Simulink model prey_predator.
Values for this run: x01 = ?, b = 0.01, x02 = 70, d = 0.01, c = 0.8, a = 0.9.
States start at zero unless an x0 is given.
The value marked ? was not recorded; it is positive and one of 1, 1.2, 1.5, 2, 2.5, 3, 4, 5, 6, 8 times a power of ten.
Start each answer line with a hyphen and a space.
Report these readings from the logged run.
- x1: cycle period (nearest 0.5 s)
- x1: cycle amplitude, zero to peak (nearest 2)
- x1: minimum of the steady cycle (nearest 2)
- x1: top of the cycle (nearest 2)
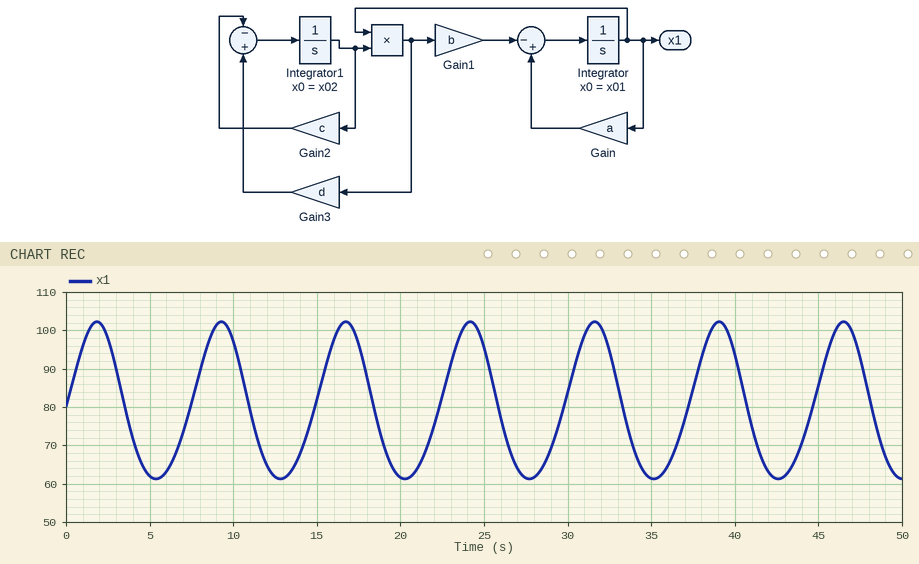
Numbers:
- 7.5 s
- 20
- 62
- 102
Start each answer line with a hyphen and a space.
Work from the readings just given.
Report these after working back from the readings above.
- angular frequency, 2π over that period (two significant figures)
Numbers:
- 0.84 rad/s
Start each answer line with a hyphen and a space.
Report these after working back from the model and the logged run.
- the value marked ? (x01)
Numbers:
- 80
